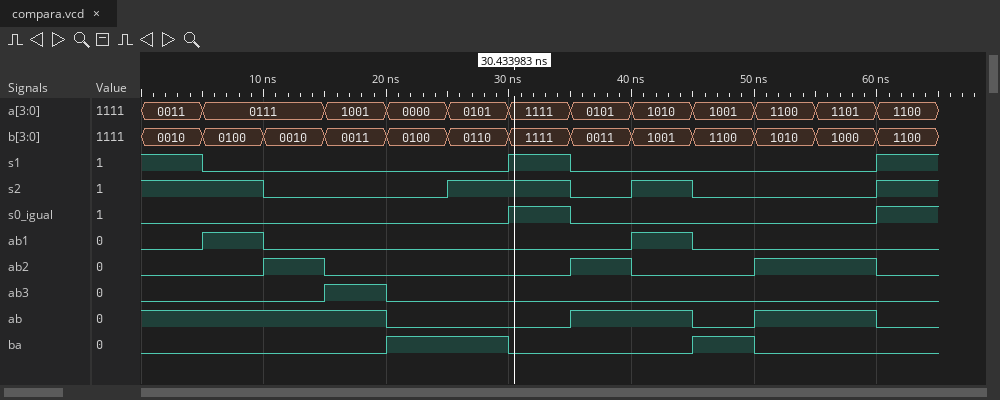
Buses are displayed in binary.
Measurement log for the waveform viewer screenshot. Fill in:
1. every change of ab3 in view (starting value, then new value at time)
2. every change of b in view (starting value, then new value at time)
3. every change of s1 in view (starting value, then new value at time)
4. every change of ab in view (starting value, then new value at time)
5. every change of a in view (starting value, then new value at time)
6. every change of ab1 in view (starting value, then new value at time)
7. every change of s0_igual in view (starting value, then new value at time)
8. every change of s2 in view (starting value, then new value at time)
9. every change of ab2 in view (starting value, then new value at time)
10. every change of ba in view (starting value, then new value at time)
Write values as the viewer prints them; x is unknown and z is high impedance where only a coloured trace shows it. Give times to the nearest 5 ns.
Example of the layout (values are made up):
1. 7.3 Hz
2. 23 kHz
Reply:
1. 0, 1 at 15 ns, 0 at 20 ns
2. 0010, 0100 at 5 ns, 0010 at 10 ns, 0011 at 15 ns, 0100 at 20 ns, 0110 at 25 ns, 1111 at 30 ns, 0011 at 35 ns, 1001 at 40 ns, 1100 at 45 ns, 1010 at 50 ns, 1000 at 55 ns, 1100 at 60 ns
3. 1, 0 at 5 ns, 1 at 30 ns, 0 at 35 ns, 1 at 60 ns
4. 1, 0 at 20 ns, 1 at 35 ns, 0 at 45 ns, 1 at 50 ns, 0 at 60 ns
5. 0011, 0111 at 5 ns, 1001 at 15 ns, 0000 at 20 ns, 0101 at 25 ns, 1111 at 30 ns, 0101 at 35 ns, 1010 at 40 ns, 1001 at 45 ns, 1100 at 50 ns, 1101 at 55 ns, 1100 at 60 ns
6. 0, 1 at 5 ns, 0 at 10 ns, 1 at 40 ns, 0 at 45 ns
7. 0, 1 at 30 ns, 0 at 35 ns, 1 at 60 ns
8. 1, 0 at 10 ns, 1 at 25 ns, 0 at 35 ns, 1 at 40 ns, 0 at 45 ns, 1 at 60 ns
9. 0, 1 at 10 ns, 0 at 15 ns, 1 at 35 ns, 0 at 40 ns, 1 at 50 ns, 0 at 60 ns
10. 0, 1 at 20 ns, 0 at 30 ns, 1 at 45 ns, 0 at 50 ns
